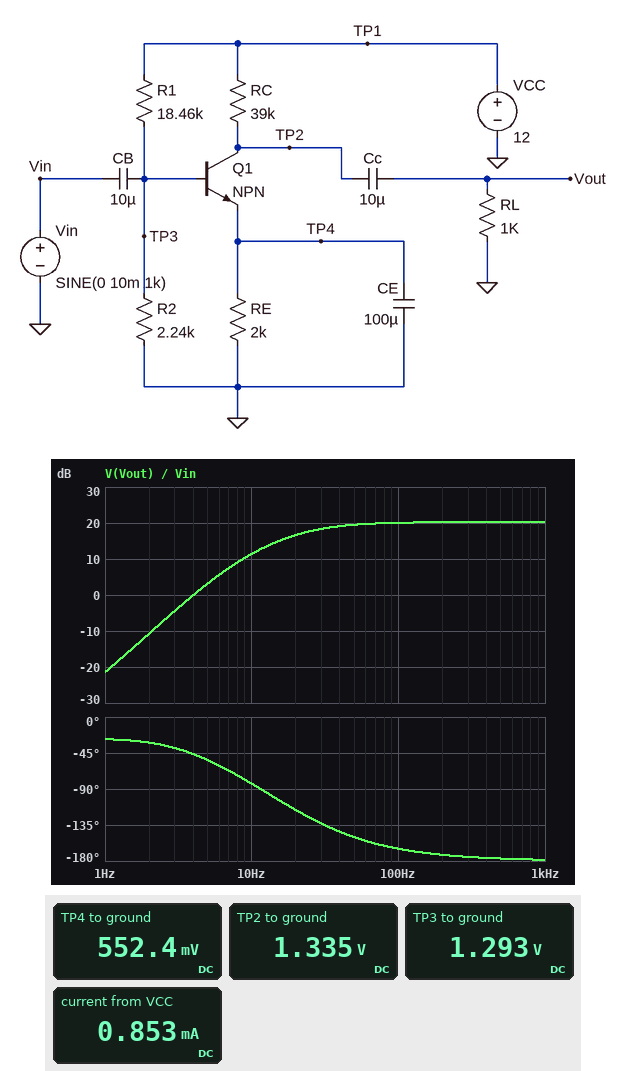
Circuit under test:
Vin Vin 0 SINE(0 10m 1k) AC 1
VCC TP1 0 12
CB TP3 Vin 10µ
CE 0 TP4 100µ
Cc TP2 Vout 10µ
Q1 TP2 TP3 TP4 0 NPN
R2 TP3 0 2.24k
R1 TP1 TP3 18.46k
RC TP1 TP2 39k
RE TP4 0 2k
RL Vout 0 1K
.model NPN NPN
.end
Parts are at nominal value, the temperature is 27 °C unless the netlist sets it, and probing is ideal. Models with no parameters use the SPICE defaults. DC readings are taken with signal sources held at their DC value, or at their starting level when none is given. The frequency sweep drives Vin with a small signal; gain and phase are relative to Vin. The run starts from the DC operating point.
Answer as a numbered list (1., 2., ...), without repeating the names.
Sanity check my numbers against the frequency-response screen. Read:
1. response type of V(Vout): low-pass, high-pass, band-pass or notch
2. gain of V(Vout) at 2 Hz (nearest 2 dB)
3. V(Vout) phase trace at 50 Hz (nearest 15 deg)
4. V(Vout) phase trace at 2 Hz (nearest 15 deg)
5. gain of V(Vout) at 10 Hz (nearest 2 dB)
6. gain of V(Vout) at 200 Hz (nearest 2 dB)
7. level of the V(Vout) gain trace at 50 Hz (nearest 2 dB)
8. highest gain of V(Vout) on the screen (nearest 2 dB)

1. high-pass
2. -10 dB
3. -150 deg
4. -30 deg
5. 12 dB
6. 20 dB
7. 20 dB
8. 20 dB
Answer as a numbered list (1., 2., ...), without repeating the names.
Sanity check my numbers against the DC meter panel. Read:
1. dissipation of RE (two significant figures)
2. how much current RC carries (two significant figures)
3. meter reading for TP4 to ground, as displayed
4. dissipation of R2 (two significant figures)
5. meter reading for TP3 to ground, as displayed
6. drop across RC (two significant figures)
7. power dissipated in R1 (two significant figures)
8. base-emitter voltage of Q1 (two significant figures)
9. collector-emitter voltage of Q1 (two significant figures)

1. 150 µW
2. 270 µA
3. 552.4 mV
4. 750 µW
5. 1.293 V
6. 11 V
7. 6.2 mW
8. 740 mV
9. 780 mV
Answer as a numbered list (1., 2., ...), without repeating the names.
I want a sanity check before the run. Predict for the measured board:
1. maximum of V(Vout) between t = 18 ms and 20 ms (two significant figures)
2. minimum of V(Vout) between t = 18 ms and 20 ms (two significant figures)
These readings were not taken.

1. 91 mV
2. -110 mV
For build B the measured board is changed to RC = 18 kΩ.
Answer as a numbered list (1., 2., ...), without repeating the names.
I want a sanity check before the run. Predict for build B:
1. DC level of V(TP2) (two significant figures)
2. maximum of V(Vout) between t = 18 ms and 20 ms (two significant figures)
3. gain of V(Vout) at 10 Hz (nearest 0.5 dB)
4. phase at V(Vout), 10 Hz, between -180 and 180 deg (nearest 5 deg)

1. 7.1 V
2. 89 mV
3. 11.0 dB
4. -80 deg
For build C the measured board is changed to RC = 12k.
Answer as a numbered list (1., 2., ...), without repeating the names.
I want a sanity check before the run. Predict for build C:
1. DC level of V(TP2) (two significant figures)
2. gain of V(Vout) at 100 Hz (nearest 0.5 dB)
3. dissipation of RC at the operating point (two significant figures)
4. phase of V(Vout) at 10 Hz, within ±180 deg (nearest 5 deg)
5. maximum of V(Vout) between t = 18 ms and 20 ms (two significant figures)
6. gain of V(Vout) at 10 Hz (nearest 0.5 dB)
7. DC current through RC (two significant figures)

1. 8.7 V
2. 19.5 dB
3. 900 µW
4. -80 deg
5. 87 mV
6. 11.0 dB
7. 270 µA
